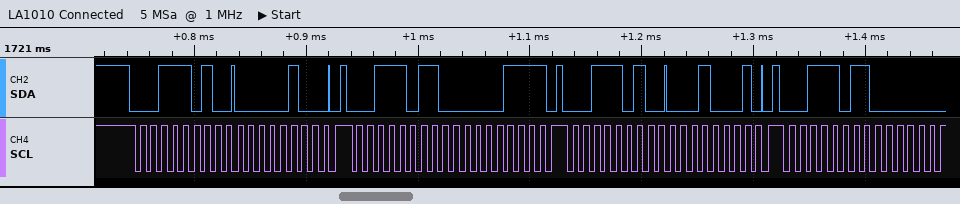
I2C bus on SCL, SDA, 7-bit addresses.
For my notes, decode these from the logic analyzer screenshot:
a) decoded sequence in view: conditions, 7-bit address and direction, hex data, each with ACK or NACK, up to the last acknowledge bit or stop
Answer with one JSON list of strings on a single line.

["start, address 1D write ACK, 04 ACK, stop, start, address 1D read ACK, 07 NACK, stop, start, address 1D write ACK, 11 ACK, stop, start, address 1D read ACK"]
